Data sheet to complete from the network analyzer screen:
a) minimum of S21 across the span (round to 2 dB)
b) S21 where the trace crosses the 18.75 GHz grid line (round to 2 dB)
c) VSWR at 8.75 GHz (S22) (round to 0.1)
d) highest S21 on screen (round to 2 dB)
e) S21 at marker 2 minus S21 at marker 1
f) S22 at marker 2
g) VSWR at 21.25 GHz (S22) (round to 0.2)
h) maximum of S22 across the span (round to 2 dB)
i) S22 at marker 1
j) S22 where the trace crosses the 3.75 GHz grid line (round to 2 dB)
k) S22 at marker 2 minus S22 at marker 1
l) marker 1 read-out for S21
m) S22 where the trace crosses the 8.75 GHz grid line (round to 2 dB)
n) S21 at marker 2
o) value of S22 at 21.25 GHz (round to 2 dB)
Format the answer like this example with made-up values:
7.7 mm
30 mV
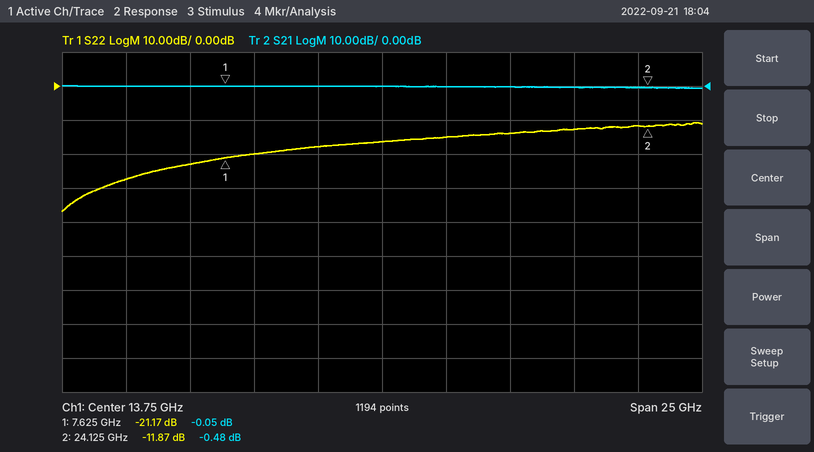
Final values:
0 dB
0 dB
1.2
0 dB
-0.43 dB
-11.87 dB
1.6
-10 dB
-21.17 dB
-28 dB
9.30 dB
-0.05 dB
-20 dB
-0.48 dB
-12 dB
